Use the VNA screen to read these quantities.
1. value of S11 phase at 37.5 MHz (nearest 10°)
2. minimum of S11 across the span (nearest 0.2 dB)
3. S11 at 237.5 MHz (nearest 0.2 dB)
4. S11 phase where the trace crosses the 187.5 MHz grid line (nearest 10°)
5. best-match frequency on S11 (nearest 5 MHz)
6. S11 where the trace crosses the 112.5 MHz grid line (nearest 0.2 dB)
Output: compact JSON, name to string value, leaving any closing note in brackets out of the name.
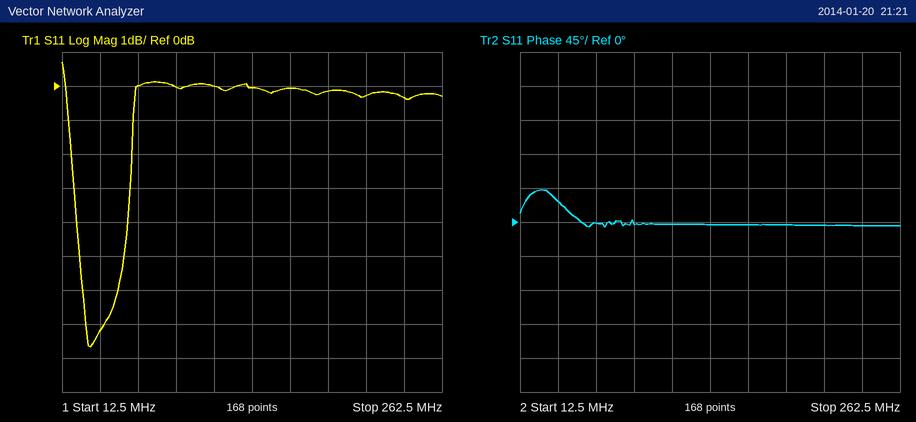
{"value of S11 phase at 37.5 MHz": "30°", "minimum of S11 across the span": "-7.6 dB", "S11 at 237.5 MHz": "-0.4 dB", "S11 phase where the trace crosses the 187.5 MHz grid line": "0°", "best-match frequency on S11": "30 MHz", "S11 where the trace crosses the 112.5 MHz grid line": "0.0 dB"}
